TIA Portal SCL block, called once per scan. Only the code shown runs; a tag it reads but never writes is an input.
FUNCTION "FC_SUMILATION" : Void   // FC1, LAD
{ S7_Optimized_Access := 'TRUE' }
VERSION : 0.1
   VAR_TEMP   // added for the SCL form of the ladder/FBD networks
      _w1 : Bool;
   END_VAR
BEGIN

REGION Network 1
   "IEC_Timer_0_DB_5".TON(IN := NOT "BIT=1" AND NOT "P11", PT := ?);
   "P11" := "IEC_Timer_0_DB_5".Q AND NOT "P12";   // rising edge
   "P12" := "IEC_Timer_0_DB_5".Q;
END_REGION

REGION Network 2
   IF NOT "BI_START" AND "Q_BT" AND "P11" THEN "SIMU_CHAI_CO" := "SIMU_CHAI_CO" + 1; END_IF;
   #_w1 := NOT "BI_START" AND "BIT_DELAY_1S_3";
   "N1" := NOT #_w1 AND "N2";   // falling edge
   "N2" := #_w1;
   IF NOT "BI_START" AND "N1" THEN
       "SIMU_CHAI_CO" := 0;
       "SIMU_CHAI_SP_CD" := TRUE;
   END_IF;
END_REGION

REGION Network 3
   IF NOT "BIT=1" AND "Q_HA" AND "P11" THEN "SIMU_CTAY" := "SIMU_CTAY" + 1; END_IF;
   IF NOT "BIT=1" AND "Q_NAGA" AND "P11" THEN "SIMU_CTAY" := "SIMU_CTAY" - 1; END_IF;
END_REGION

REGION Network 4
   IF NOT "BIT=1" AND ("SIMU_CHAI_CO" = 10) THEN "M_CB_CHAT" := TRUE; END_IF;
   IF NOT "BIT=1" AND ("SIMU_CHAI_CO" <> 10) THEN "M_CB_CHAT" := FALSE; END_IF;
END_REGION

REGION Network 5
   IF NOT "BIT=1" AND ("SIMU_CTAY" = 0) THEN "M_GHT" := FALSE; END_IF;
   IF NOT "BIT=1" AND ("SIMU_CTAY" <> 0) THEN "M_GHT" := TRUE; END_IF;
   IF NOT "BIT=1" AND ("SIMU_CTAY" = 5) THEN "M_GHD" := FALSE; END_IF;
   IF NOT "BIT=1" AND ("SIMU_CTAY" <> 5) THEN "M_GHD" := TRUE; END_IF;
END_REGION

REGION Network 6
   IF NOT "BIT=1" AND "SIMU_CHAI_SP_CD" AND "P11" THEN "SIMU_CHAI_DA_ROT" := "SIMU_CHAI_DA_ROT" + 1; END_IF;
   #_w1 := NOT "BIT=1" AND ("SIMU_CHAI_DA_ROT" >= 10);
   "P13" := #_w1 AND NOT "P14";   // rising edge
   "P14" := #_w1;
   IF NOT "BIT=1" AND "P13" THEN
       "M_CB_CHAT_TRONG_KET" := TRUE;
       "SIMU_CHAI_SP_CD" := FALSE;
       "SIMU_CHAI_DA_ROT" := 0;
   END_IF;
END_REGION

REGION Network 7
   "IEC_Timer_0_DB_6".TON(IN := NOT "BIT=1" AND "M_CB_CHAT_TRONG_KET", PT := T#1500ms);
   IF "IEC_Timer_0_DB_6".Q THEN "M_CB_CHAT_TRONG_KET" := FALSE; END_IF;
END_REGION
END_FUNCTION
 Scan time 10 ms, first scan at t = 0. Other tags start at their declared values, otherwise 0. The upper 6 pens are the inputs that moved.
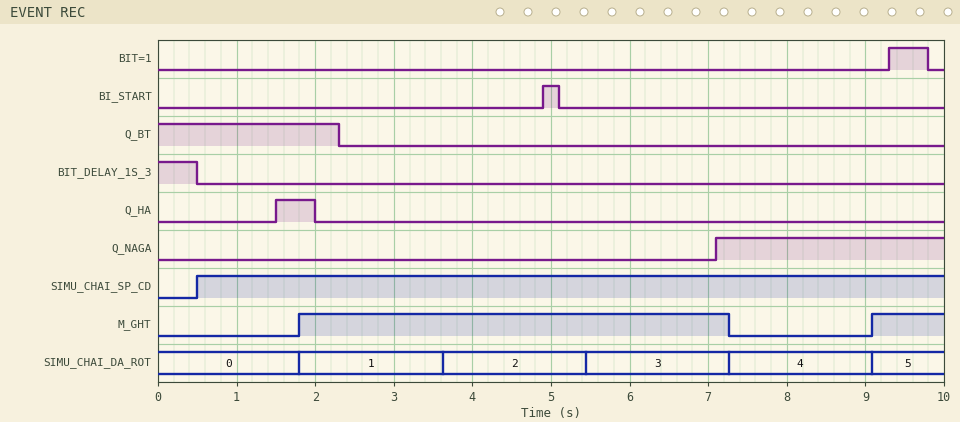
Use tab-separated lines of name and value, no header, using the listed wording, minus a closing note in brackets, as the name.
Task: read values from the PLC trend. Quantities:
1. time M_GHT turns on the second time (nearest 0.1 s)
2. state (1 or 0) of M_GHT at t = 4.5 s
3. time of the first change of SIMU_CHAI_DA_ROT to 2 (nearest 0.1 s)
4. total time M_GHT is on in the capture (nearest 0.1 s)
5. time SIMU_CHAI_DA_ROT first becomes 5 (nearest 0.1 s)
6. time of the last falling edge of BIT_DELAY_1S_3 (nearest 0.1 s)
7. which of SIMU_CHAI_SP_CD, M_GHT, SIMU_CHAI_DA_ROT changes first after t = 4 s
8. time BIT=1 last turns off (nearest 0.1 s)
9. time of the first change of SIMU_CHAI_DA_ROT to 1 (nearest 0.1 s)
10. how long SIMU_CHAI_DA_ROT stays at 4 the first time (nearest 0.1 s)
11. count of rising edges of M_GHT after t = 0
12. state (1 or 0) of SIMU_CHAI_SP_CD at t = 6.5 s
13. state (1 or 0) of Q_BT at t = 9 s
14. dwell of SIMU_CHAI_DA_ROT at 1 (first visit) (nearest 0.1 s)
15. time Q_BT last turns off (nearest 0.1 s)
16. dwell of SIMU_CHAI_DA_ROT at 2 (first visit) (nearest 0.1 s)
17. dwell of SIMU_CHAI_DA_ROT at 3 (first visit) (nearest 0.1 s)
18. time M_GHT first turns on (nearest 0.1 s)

time M_GHT turns on the second time	9.1 s
state (1 or 0) of M_GHT at t = 4.5 s	1
time of the first change of SIMU_CHAI_DA_ROT to 2	3.6 s
total time M_GHT is on in the capture	6.4 s
time SIMU_CHAI_DA_ROT first becomes 5	9.1 s
time of the last falling edge of BIT_DELAY_1S_3	0.5 s
which of SIMU_CHAI_SP_CD, M_GHT, SIMU_CHAI_DA_ROT changes first after t = 4 s	SIMU_CHAI_DA_ROT
time BIT=1 last turns off	9.8 s
time of the first change of SIMU_CHAI_DA_ROT to 1	1.8 s
how long SIMU_CHAI_DA_ROT stays at 4 the first time	1.8 s
count of rising edges of M_GHT after t = 0	2
state (1 or 0) of SIMU_CHAI_SP_CD at t = 6.5 s	1
state (1 or 0) of Q_BT at t = 9 s	0
dwell of SIMU_CHAI_DA_ROT at 1 (first visit)	1.8 s
time Q_BT last turns off	2.3 s
dwell of SIMU_CHAI_DA_ROT at 2 (first visit)	1.8 s
dwell of SIMU_CHAI_DA_ROT at 3 (first visit)	1.8 s
time M_GHT first turns on	1.8 s
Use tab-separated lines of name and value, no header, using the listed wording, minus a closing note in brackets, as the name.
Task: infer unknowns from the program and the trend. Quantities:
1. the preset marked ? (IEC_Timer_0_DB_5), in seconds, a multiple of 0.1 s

the preset marked ? (IEC_Timer_0_DB_5), in seconds, a multiple of 0.1 s	1.8 s
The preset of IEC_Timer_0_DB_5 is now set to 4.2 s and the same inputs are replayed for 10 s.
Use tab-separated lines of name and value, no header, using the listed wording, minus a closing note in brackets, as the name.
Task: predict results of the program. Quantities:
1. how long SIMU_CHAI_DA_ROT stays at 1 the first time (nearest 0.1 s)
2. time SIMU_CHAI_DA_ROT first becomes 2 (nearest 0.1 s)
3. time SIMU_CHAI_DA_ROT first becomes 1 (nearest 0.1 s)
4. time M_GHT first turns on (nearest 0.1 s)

how long SIMU_CHAI_DA_ROT stays at 1 the first time	4.2 s
time SIMU_CHAI_DA_ROT first becomes 2	8.4 s
time SIMU_CHAI_DA_ROT first becomes 1	4.2 s
time M_GHT first turns on	8.4 s
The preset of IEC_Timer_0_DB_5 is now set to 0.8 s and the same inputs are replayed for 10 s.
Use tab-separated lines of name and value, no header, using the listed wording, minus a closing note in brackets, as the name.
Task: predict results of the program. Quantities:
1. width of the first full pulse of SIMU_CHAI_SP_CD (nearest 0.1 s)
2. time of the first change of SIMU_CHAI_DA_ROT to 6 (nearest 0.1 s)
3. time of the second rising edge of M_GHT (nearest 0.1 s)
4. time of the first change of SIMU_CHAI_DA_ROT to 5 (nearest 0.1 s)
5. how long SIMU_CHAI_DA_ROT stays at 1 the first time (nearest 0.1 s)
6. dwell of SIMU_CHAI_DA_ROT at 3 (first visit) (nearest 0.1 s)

width of the first full pulse of SIMU_CHAI_SP_CD	7.7 s
time of the first change of SIMU_CHAI_DA_ROT to 6	4.9 s
time of the second rising edge of M_GHT	8.2 s
time of the first change of SIMU_CHAI_DA_ROT to 5	4.1 s
how long SIMU_CHAI_DA_ROT stays at 1 the first time	0.8 s
dwell of SIMU_CHAI_DA_ROT at 3 (first visit)	0.8 s
